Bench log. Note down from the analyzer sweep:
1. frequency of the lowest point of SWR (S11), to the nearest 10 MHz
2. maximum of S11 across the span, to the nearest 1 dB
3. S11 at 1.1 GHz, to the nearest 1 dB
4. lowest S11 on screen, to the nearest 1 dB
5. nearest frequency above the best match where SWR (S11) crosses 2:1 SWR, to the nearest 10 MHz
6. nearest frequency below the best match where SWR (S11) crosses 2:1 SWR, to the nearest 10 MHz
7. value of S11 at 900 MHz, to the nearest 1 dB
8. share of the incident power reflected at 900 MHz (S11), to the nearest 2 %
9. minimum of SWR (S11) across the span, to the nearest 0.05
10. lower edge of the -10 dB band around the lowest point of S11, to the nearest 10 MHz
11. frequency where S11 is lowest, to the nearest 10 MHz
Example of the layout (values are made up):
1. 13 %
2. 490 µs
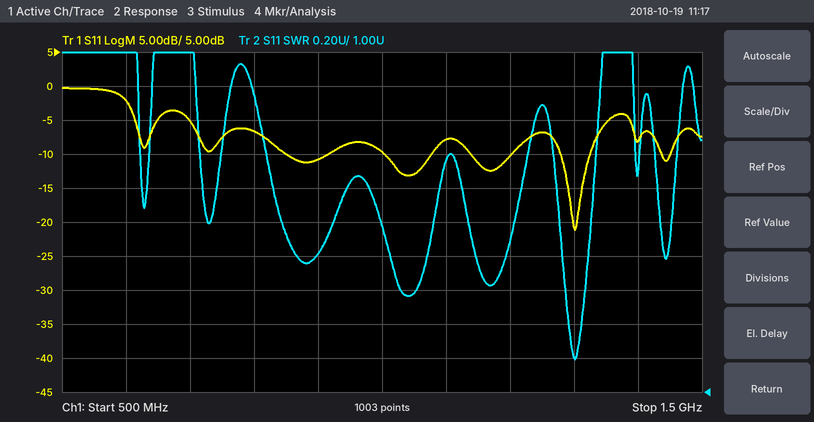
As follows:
1. 1.30 GHz
2. 0 dB
3. -8 dB
4. -21 dB
5. 1.33 GHz
6. 1.28 GHz
7. -11 dB
8. 8 %
9. 1.20
10. 1.28 GHz
11. 1.30 GHz
